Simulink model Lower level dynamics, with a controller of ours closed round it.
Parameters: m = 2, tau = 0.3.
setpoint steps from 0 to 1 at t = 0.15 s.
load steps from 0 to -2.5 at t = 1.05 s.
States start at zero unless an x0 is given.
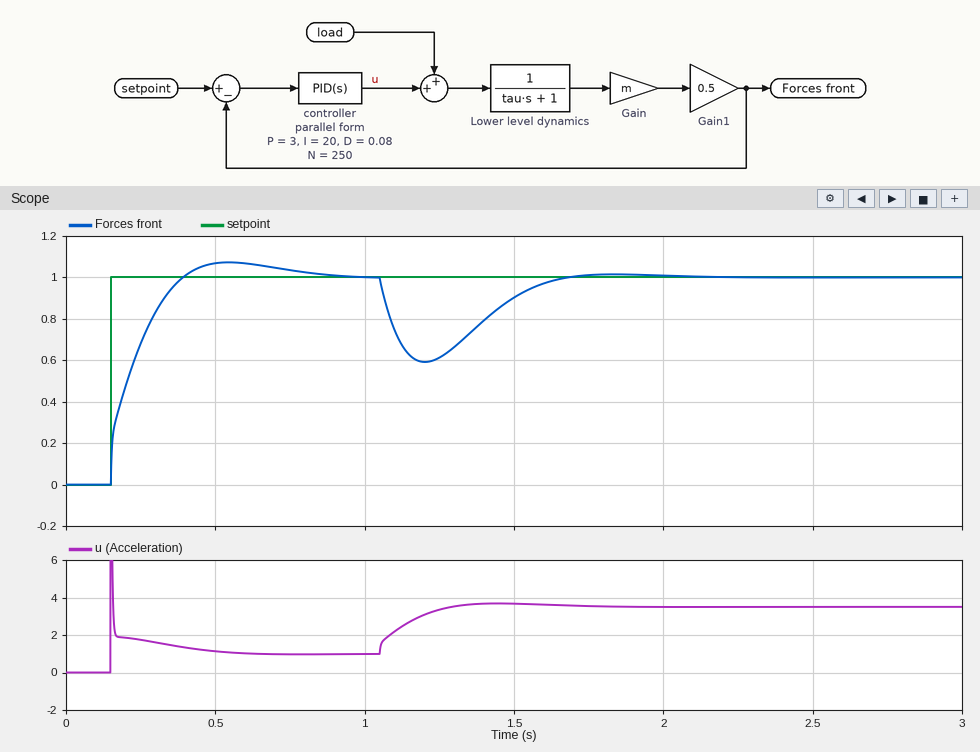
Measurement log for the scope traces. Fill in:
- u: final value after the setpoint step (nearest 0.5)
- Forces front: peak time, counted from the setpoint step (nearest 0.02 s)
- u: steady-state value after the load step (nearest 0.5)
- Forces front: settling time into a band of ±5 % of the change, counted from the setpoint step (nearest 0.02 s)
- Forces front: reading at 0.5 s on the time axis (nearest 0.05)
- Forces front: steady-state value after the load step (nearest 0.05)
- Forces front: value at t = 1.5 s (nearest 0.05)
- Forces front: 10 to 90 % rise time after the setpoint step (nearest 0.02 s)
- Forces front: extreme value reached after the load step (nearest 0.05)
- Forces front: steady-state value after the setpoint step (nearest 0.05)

1.0
0.40 s
3.5
0.54 s
1.05
1.00
0.90
0.18 s
0.60
1.00
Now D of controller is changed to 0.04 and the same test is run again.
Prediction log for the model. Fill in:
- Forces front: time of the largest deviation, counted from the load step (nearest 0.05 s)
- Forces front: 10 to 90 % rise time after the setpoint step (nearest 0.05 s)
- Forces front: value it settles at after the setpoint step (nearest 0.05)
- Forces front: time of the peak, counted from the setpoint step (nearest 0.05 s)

0.15 s
0.15 s
1.00
0.35 s
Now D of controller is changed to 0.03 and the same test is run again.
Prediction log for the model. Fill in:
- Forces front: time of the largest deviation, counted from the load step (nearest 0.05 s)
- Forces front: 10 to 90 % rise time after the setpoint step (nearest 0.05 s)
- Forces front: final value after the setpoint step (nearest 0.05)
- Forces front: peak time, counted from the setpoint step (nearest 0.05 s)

0.15 s
0.15 s
1.00
0.35 s
